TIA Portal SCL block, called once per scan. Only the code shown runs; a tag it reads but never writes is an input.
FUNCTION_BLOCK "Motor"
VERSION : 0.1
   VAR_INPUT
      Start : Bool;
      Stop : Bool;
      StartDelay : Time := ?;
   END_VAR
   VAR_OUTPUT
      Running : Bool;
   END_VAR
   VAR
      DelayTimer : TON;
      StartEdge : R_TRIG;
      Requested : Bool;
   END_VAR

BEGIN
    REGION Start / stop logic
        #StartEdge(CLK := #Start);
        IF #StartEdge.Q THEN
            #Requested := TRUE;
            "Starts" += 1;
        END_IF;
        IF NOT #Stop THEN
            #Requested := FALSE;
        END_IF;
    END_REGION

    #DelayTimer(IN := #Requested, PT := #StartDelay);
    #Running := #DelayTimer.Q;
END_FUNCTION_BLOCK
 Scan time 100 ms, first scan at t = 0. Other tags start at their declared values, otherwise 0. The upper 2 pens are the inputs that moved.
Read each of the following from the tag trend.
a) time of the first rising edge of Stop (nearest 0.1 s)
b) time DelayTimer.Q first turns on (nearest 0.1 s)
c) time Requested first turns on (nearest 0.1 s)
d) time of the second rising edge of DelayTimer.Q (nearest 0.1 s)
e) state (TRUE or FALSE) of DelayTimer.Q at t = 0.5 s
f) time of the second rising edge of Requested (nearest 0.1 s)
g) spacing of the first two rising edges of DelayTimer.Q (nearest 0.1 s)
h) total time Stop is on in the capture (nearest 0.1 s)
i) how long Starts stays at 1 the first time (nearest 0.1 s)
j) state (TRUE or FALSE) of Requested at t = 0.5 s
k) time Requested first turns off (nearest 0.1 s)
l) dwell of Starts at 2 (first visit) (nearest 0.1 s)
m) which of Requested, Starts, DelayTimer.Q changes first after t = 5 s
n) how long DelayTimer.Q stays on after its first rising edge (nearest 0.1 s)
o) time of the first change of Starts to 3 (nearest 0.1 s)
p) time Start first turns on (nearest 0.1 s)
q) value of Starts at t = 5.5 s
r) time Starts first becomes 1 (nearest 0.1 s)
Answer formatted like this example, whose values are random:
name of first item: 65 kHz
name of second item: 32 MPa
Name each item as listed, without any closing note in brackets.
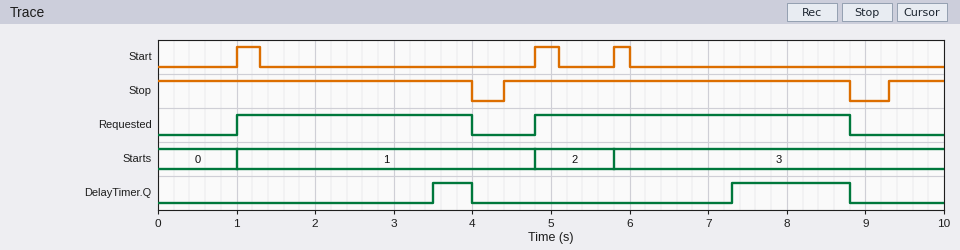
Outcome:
time of the first rising edge of Stop: 4.4 s
time DelayTimer.Q first turns on: 3.5 s
time Requested first turns on: 1.0 s
time of the second rising edge of DelayTimer.Q: 7.3 s
state (TRUE or FALSE) of DelayTimer.Q at t = 0.5 s: FALSE
time of the second rising edge of Requested: 4.8 s
spacing of the first two rising edges of DelayTimer.Q: 3.8 s
total time Stop is on in the capture: 9.1 s
how long Starts stays at 1 the first time: 3.8 s
state (TRUE or FALSE) of Requested at t = 0.5 s: FALSE
time Requested first turns off: 4.0 s
dwell of Starts at 2 (first visit): 1.0 s
which of Requested, Starts, DelayTimer.Q changes first after t = 5 s: Starts
how long DelayTimer.Q stays on after its first rising edge: 0.5 s
time of the first change of Starts to 3: 5.8 s
time Start first turns on: 1.0 s
value of Starts at t = 5.5 s: 2
time Starts first becomes 1: 1.0 s
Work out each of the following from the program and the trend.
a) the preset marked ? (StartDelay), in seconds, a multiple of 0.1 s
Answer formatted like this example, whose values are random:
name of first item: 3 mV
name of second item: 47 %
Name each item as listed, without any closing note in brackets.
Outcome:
the preset marked ? (StartDelay), in seconds, a multiple of 0.1 s: 2.5 s
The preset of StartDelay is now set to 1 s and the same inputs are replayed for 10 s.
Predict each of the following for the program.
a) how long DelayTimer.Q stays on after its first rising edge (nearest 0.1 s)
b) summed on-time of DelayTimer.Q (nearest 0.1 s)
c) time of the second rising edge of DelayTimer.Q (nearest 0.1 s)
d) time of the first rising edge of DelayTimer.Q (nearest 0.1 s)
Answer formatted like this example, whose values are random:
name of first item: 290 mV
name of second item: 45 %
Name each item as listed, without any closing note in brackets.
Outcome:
how long DelayTimer.Q stays on after its first rising edge: 2.0 s
summed on-time of DelayTimer.Q: 5.0 s
time of the second rising edge of DelayTimer.Q: 5.8 s
time of the first rising edge of DelayTimer.Q: 2.0 s
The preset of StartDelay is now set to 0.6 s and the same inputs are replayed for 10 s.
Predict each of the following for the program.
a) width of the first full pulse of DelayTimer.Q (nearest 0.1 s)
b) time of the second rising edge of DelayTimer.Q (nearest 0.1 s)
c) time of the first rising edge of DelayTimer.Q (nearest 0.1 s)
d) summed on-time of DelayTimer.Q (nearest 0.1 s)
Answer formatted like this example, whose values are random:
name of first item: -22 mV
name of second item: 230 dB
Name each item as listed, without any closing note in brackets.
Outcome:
width of the first full pulse of DelayTimer.Q: 2.4 s
time of the second rising edge of DelayTimer.Q: 5.4 s
time of the first rising edge of DelayTimer.Q: 1.6 s
summed on-time of DelayTimer.Q: 5.8 s
